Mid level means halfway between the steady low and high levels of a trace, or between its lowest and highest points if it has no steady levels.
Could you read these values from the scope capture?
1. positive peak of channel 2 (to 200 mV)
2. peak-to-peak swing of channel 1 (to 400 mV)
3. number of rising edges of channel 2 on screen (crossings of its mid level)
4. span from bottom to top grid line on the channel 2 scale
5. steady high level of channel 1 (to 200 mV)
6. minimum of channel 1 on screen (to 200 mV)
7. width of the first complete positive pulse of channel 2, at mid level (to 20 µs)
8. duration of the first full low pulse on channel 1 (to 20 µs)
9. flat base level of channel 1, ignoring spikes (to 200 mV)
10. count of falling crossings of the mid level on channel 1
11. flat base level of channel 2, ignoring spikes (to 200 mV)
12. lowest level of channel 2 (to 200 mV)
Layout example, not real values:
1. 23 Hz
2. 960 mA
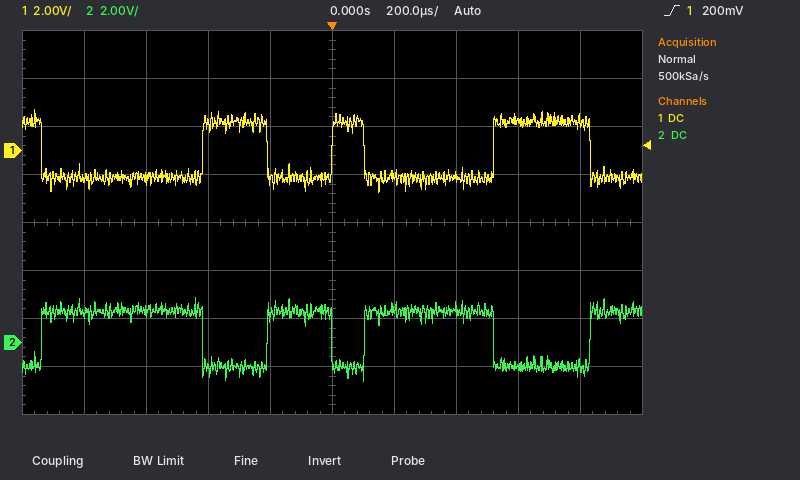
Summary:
1. 1.8 V
2. 3.6 V
3. 4
4. 16 V
5. 1.2 V
6. -1.8 V
7. 520 µs
8. 520 µs
9. -1.2 V
10. 4
11. -1.0 V
12. -1.6 V
